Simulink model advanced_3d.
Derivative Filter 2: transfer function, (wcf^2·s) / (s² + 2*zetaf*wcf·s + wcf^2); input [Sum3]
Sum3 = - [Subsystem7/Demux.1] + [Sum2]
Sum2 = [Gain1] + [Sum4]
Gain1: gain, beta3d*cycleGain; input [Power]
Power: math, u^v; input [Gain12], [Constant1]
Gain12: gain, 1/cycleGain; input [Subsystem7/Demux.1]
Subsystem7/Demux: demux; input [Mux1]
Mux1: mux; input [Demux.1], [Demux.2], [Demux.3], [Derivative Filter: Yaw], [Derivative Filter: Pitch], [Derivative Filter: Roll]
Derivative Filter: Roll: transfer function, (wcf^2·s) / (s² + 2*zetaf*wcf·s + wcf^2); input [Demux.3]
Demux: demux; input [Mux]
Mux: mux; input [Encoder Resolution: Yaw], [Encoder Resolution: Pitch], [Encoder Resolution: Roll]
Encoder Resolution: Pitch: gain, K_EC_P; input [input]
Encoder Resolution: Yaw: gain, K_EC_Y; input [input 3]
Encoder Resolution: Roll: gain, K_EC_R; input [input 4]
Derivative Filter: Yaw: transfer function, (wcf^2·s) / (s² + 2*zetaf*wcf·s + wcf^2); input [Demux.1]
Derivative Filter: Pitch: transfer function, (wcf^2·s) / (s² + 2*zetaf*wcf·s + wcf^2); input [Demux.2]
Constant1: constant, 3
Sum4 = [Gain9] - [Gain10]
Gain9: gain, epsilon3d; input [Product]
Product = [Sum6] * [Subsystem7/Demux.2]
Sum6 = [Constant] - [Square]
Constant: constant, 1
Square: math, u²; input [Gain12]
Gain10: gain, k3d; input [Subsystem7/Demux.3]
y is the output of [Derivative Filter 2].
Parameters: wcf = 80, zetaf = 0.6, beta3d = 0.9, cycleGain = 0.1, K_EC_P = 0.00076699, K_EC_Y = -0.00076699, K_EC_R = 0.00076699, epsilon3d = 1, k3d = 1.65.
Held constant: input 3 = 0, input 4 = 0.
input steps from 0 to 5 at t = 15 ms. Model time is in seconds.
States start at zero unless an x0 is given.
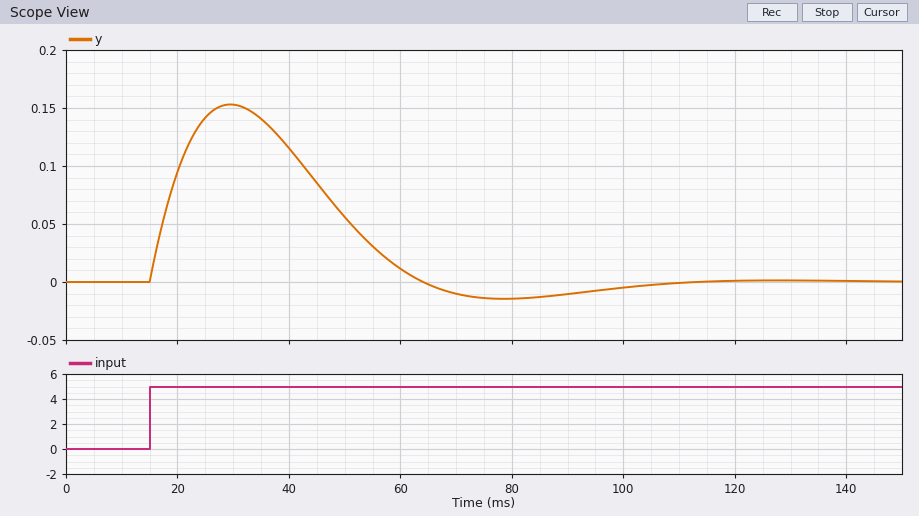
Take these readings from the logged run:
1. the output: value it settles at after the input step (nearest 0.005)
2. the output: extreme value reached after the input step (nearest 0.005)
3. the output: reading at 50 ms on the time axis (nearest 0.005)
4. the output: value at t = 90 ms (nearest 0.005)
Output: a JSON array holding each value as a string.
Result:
["0.000", "0.155", "0.055", "-0.010"]
